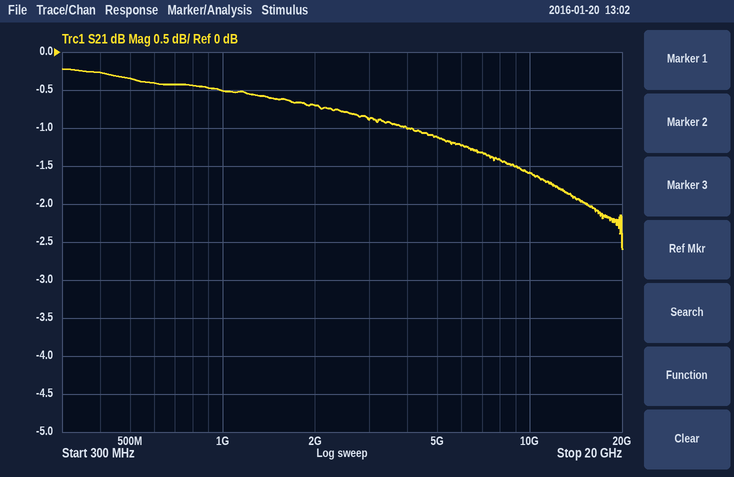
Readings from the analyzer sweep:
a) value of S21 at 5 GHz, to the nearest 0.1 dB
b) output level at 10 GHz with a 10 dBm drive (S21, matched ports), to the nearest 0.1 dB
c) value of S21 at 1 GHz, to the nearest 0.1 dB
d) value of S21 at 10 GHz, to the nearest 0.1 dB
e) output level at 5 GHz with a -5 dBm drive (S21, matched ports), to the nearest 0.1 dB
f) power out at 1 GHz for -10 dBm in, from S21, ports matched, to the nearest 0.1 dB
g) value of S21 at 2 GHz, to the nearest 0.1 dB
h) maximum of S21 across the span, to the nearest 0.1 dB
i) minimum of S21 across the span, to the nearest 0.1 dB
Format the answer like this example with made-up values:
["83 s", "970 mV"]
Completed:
["-1.1 dB", "8.4 dBm", "-0.5 dB", "-1.6 dB", "-6.1 dBm", "-10.5 dBm", "-0.7 dB", "-0.2 dB", "-2.6 dB"]
